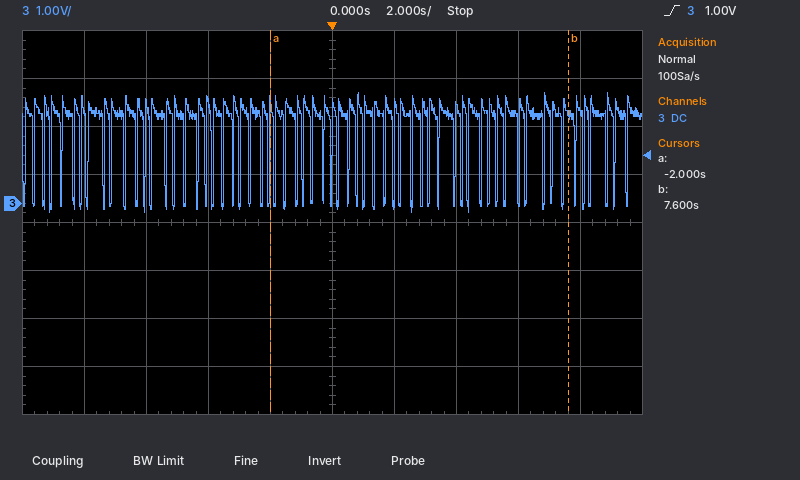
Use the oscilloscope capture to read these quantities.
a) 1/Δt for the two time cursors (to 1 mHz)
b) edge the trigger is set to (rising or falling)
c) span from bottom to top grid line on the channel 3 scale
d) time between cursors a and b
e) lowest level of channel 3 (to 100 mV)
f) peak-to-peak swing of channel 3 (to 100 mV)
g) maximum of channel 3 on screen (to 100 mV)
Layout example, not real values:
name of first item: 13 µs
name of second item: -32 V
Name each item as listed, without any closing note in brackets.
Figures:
1/Δt for the two time cursors: 104 mHz
edge the trigger is set to: rising
span from bottom to top grid line on the channel 3 scale: 8 V
time between cursors a and b: 9.6 s
lowest level of channel 3: -200 mV
peak-to-peak swing of channel 3: 2.5 V
maximum of channel 3 on screen: 2.3 V
